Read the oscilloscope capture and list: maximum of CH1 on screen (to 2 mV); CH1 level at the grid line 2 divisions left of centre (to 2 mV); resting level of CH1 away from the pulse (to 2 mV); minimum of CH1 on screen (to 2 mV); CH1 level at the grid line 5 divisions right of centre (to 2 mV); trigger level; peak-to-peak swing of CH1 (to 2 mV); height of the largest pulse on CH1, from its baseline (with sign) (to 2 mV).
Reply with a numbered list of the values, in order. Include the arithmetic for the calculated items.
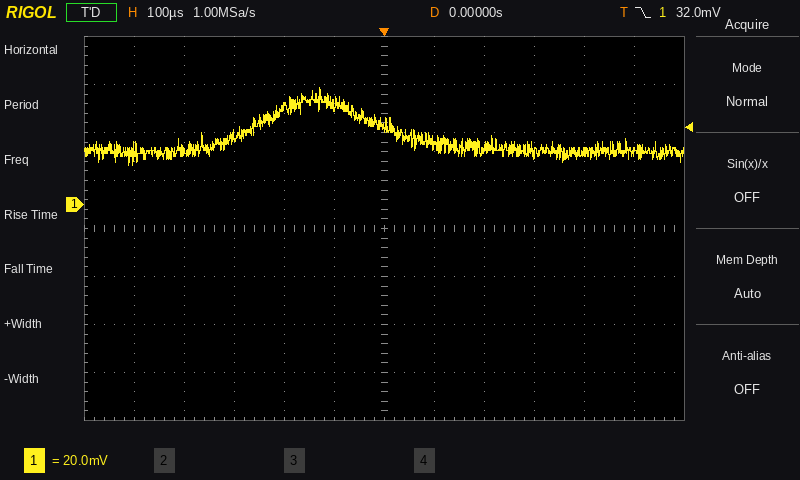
1. 48 mV
2. 40 mV
3. 22 mV
4. 16 mV
5. 22 mV
6. 32.0 mV
7. 48 mV − (16 mV) = 32 mV
8. 48 mV − (22 mV) = +26 mV
